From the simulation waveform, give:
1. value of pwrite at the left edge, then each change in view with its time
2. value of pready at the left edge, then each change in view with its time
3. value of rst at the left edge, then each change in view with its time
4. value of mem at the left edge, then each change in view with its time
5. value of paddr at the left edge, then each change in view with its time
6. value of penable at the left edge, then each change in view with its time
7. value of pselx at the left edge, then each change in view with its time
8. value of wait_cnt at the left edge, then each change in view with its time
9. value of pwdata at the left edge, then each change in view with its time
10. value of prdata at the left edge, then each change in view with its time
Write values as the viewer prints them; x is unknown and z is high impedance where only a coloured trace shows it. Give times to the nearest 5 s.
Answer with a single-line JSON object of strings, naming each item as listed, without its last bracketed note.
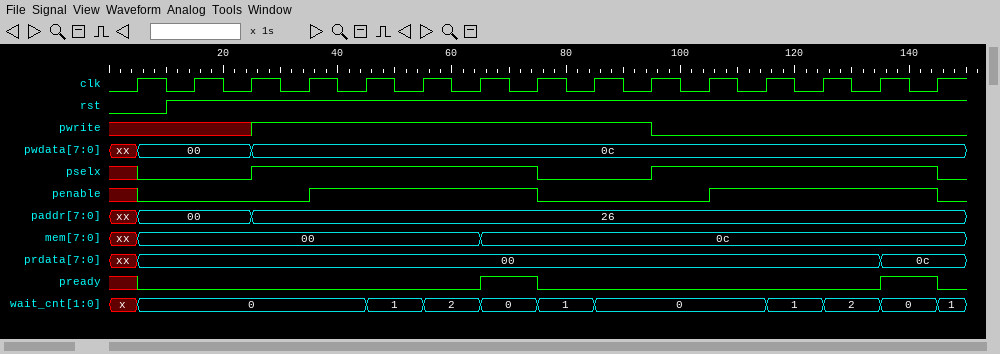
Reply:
{"value of pwrite at the left edge, then each change in view with its time": "x, 1 at 25 s, 0 at 95 s", "value of pready at the left edge, then each change in view with its time": "x, 0 at 5 s, 1 at 65 s, 0 at 75 s, 1 at 135 s, 0 at 145 s", "value of rst at the left edge, then each change in view with its time": "0, 1 at 10 s", "value of mem at the left edge, then each change in view with its time": "xx, 00 at 5 s, 0c at 65 s", "value of paddr at the left edge, then each change in view with its time": "xx, 00 at 5 s, 26 at 25 s", "value of penable at the left edge, then each change in view with its time": "x, 0 at 5 s, 1 at 35 s, 0 at 75 s, 1 at 105 s, 0 at 145 s", "value of pselx at the left edge, then each change in view with its time": "x, 0 at 5 s, 1 at 25 s, 0 at 75 s, 1 at 95 s, 0 at 145 s", "value of wait_cnt at the left edge, then each change in view with its time": "x, 0 at 5 s, 1 at 45 s, 2 at 55 s, 0 at 65 s, 1 at 75 s, 0 at 85 s, 1 at 115 s, 2 at 125 s, 0 at 135 s, 1 at 145 s", "value of pwdata at the left edge, then each change in view with its time": "xx, 00 at 5 s, 0c at 25 s", "value of prdata at the left edge, then each change in view with its time": "xx, 00 at 5 s, 0c at 135 s"}
